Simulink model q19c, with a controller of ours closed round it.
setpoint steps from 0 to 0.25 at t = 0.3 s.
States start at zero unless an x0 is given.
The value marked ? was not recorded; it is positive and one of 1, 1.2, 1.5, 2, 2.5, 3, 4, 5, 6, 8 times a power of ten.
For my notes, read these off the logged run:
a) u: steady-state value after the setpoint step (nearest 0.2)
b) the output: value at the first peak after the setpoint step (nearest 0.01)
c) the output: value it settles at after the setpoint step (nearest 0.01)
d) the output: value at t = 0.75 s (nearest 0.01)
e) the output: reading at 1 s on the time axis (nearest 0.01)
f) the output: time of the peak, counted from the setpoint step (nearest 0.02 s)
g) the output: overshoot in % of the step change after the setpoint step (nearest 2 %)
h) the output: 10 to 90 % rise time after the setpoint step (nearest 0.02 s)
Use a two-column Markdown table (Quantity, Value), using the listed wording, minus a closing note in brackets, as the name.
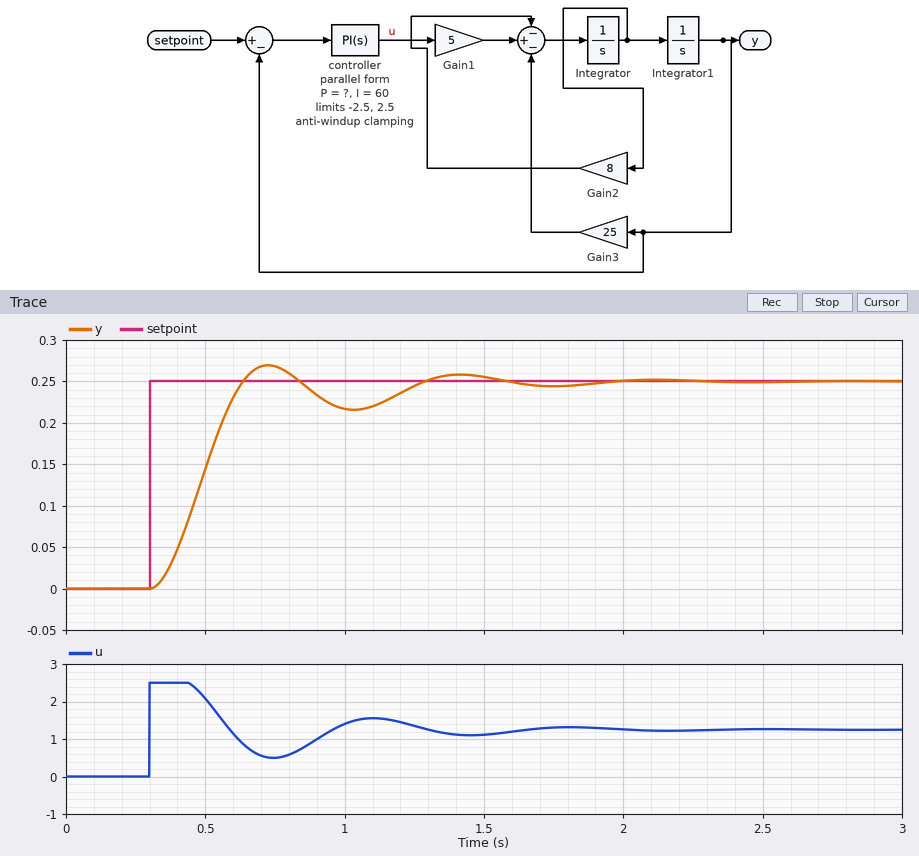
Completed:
| Quantity | Value |
|---|---|
| u: steady-state value after the setpoint step | 1.2 |
| the output: value at the first peak after the setpoint step | 0.27 |
| the output: value it settles at after the setpoint step | 0.25 |
| the output: value at t = 0.75 s | 0.27 |
| the output: reading at 1 s on the time axis | 0.22 |
| the output: time of the peak, counted from the setpoint step | 0.42 s |
| the output: overshoot in % of the step change after the setpoint step | 8 % |
| the output: 10 to 90 % rise time after the setpoint step | 0.22 s |
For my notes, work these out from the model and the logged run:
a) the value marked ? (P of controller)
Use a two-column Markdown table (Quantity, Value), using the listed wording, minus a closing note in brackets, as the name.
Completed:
| Quantity | Value |
|---|---|
| the value marked ? | 15 |
